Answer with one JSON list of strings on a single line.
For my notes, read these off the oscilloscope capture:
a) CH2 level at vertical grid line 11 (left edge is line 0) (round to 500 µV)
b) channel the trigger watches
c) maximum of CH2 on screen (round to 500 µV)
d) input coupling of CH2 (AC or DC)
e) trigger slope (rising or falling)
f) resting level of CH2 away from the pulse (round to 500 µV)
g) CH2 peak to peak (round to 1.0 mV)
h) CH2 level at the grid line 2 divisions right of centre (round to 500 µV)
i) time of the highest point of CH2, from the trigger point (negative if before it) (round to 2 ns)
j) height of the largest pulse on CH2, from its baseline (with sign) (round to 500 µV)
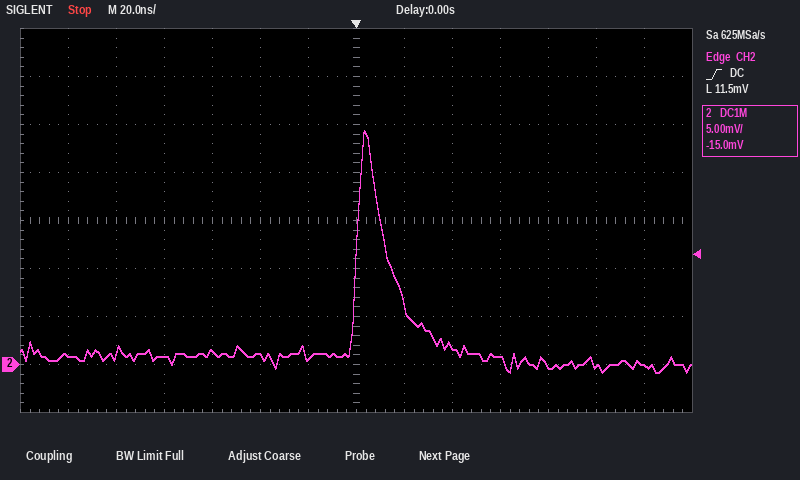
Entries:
["0.0 mV", "CH2", "24.5 mV", "DC", "rising", "1.0 mV", "25.0 mV", "2.0 mV", "+4 ns", "+23.5 mV"]
